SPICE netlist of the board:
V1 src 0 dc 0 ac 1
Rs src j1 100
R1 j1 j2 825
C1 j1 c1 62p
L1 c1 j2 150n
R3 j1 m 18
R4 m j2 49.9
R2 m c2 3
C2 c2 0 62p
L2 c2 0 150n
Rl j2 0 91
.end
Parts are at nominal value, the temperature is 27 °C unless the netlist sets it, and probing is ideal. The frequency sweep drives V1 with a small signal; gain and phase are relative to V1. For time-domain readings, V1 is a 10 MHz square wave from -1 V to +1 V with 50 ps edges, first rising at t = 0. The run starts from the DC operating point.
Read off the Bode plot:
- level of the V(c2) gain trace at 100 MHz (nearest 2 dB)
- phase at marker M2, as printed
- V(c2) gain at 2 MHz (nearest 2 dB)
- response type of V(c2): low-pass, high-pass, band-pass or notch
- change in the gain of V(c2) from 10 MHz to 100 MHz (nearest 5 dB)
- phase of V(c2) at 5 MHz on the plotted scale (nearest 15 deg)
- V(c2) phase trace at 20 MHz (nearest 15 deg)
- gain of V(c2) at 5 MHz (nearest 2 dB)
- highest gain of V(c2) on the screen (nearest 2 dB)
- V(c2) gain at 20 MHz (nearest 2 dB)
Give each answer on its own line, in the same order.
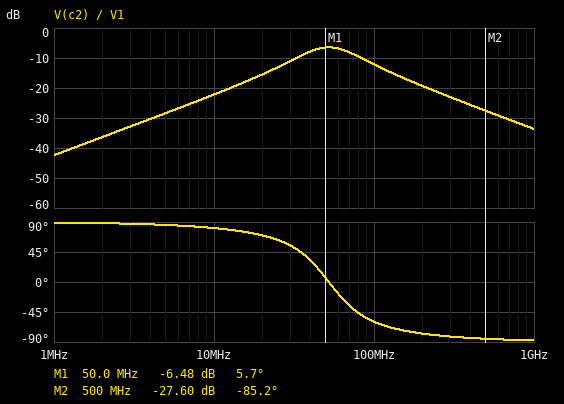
-12 dB
-85.2 deg
-36 dB
band-pass
10 dB
90 deg
75 deg
-28 dB
-6 dB
-16 dB
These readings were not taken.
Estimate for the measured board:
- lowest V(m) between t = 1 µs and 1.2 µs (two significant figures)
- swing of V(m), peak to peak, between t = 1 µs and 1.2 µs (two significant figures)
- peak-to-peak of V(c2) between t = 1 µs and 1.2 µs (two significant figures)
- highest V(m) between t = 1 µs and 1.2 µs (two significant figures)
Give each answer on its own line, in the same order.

-480 mV
950 mV
950 mV
480 mV
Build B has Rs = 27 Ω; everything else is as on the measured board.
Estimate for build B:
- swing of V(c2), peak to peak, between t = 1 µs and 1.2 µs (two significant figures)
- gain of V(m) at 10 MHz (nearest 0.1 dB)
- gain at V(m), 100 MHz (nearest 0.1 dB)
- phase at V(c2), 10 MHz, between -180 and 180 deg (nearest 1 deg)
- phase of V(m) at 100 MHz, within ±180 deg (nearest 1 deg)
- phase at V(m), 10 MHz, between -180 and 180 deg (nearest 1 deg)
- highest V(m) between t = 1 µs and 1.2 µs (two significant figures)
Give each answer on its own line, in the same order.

1.9 V
-13.9 dB
-5.6 dB
75 deg
-42 deg
58 deg
940 mV
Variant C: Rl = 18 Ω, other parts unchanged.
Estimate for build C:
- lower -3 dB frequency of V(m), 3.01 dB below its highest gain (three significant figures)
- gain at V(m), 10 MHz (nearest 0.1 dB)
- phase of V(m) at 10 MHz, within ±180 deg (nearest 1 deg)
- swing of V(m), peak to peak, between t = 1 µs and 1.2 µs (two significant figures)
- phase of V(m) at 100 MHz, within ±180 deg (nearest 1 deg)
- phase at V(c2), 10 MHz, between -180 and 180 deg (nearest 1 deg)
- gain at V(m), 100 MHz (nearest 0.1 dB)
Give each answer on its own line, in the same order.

22.0 MHz
-22.1 dB
58 deg
670 mV
-34 deg
75 deg
-13.2 dB
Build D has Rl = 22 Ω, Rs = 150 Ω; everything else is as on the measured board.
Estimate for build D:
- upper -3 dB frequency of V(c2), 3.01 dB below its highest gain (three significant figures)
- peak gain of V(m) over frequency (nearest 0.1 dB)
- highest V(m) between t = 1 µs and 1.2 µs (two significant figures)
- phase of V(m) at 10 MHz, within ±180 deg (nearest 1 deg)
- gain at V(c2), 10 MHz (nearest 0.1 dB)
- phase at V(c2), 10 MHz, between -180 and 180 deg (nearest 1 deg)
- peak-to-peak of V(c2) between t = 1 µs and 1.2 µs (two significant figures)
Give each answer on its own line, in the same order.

118 MHz
-14.3 dB
250 mV
60 deg
-25.4 dB
77 deg
520 mV
